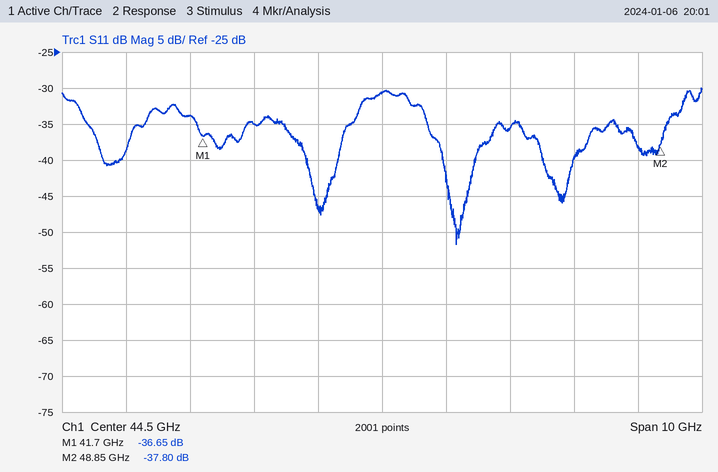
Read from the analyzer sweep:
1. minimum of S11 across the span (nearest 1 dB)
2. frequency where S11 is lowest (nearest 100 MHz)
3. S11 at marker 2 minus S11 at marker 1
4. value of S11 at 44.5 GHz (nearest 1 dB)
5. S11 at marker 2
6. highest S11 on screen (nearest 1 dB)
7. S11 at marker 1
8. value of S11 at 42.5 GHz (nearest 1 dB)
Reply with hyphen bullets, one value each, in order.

- -52 dB
- 45.7 GHz
- -1.15 dB
- -31 dB
- -37.80 dB
- -30 dB
- -36.65 dB
- -35 dB
